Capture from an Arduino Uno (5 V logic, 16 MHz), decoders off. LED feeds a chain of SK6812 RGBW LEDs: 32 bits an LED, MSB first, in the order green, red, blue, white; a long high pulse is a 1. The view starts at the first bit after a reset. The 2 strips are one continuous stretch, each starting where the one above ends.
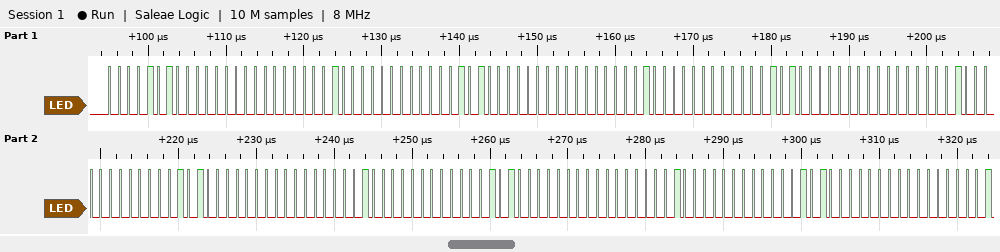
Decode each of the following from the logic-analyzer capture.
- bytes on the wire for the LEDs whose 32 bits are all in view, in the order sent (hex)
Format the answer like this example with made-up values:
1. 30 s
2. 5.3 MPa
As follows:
1. 0A 00 01 00 0A 00 01 00 0A 00 01 00 0A 00 01 00 0A 00 01 00
